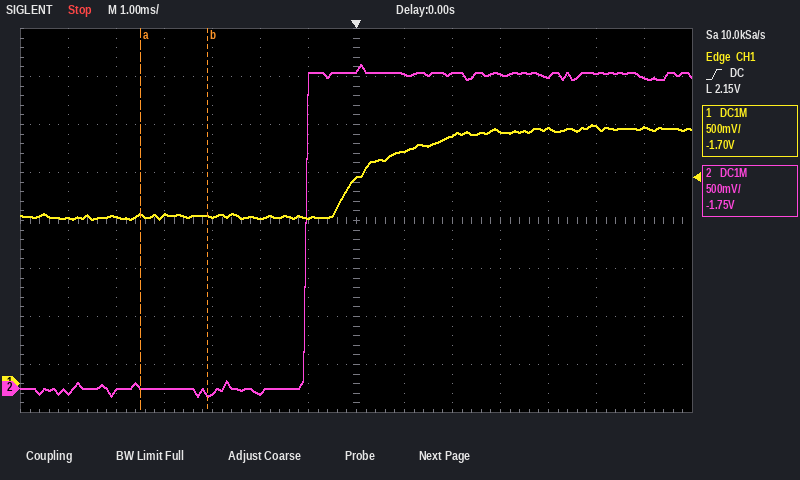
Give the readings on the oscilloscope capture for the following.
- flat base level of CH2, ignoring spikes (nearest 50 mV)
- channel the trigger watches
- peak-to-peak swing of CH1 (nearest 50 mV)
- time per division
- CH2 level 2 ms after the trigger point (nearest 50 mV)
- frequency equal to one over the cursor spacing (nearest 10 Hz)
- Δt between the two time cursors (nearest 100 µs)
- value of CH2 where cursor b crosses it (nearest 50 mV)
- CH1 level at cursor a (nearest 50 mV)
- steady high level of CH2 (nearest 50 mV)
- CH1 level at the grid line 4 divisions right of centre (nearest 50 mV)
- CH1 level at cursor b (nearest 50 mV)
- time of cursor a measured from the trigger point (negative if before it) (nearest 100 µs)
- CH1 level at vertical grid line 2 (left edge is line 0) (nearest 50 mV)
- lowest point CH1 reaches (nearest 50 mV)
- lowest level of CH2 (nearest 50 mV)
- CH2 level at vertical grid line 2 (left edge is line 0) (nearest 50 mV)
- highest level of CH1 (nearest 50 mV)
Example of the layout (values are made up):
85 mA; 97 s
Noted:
0 mV; CH1; 1.00 V; 1 ms; 3.30 V; 710 Hz; 1.4 ms; -50 mV; 1.75 V; 3.30 V; 2.65 V; 1.75 V; -4.5 ms; 1.75 V; 1.70 V; -100 mV; 0 mV; 2.70 V
